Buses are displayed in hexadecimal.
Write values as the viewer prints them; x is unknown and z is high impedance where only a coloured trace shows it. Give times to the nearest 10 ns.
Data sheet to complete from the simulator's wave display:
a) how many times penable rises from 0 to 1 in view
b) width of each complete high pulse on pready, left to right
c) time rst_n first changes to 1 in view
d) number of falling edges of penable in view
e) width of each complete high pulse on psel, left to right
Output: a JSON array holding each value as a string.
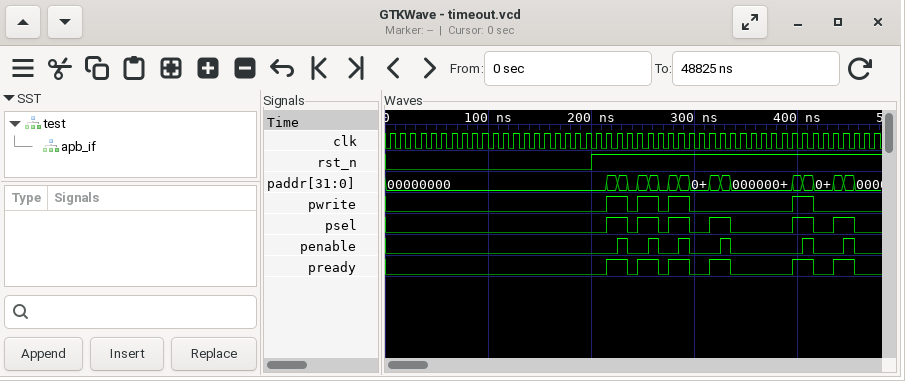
["6", "20 ns, 20 ns, 20 ns, 20 ns, 20 ns, 20 ns", "200 ns", "6", "20 ns, 20 ns, 20 ns, 20 ns, 20 ns, 20 ns"]
